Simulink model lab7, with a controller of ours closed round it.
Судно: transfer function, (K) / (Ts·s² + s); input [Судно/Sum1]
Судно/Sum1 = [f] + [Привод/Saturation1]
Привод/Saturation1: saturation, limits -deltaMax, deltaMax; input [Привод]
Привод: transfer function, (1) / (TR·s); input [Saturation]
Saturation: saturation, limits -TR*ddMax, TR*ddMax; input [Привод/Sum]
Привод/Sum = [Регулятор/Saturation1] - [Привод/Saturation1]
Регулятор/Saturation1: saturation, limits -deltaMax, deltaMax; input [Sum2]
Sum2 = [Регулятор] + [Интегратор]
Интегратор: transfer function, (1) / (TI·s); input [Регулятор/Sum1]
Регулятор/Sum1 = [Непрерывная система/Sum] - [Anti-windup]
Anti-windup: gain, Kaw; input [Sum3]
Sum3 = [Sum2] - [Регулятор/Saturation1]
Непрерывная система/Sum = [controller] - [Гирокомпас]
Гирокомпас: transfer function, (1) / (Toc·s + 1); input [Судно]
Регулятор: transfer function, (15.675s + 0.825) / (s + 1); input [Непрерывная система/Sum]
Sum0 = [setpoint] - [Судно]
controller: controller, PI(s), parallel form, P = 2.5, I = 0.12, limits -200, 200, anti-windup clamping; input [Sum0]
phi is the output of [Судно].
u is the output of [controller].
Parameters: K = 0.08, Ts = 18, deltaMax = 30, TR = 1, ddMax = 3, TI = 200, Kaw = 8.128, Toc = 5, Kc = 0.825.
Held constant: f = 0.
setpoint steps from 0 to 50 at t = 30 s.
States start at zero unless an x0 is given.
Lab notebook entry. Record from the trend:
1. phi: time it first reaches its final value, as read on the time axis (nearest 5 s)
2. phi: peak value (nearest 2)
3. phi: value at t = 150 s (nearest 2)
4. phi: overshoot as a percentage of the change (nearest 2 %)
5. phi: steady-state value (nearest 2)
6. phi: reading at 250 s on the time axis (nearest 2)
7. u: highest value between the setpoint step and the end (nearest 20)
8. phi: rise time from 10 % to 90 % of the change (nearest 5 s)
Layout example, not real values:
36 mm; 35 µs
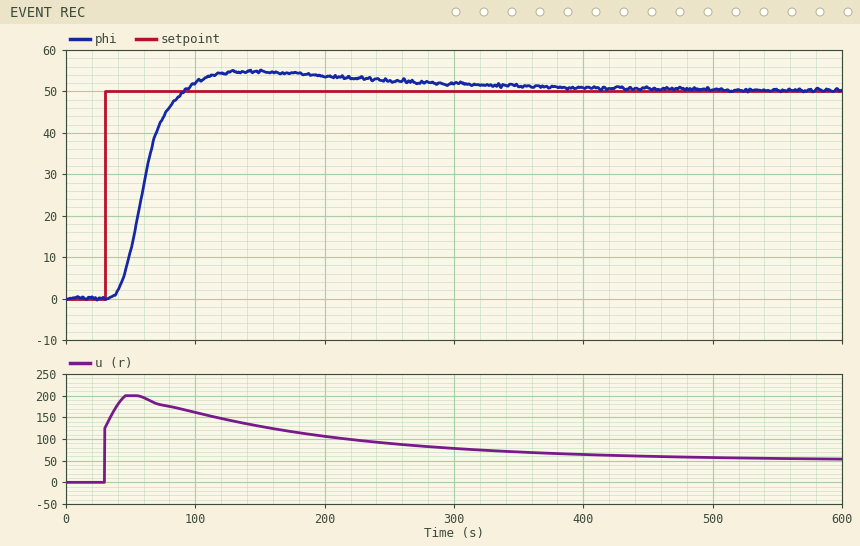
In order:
90 s; 54; 54; 10 %; 50; 52; 200; 35 s
